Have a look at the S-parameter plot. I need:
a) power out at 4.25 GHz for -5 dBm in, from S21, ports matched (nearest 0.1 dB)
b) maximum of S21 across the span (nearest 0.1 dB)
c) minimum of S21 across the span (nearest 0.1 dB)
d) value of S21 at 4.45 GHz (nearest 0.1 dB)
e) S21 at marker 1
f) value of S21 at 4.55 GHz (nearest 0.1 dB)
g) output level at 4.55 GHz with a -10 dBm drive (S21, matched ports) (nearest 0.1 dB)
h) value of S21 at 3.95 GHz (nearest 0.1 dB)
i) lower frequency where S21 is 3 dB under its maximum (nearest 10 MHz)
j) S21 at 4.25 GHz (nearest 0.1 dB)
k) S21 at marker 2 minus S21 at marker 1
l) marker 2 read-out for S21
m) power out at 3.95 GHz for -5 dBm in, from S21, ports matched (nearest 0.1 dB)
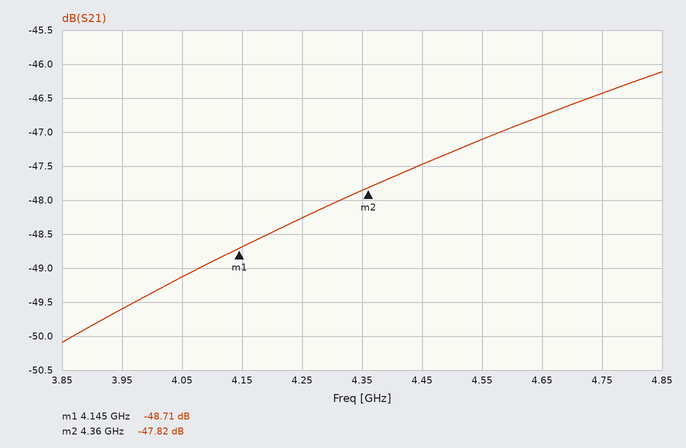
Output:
-53.3 dBm
-46.1 dB
-50.1 dB
-47.5 dB
-48.71 dB
-47.1 dB
-57.1 dBm
-49.6 dB
4.05 GHz
-48.3 dB
0.89 dB
-47.82 dB
-54.6 dBm
